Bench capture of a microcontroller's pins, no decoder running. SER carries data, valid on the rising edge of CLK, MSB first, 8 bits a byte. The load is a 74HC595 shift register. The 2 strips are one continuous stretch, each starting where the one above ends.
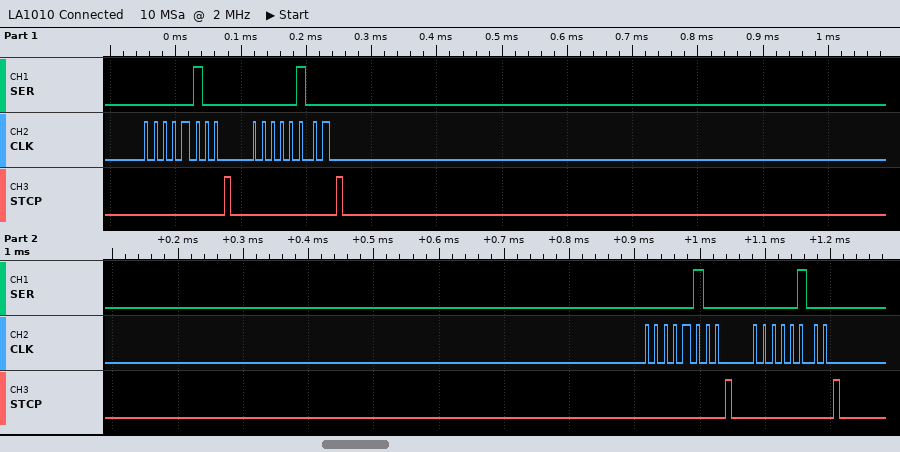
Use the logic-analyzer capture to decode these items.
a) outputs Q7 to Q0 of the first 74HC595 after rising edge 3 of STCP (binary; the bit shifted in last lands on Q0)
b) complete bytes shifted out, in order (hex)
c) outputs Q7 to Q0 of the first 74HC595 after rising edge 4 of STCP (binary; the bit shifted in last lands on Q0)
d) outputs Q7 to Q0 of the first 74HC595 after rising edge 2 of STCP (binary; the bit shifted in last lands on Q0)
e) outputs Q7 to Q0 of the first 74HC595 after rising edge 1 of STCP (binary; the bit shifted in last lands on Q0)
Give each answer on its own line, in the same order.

00000100
04 04 04 04
00000100
00000100
00000100
